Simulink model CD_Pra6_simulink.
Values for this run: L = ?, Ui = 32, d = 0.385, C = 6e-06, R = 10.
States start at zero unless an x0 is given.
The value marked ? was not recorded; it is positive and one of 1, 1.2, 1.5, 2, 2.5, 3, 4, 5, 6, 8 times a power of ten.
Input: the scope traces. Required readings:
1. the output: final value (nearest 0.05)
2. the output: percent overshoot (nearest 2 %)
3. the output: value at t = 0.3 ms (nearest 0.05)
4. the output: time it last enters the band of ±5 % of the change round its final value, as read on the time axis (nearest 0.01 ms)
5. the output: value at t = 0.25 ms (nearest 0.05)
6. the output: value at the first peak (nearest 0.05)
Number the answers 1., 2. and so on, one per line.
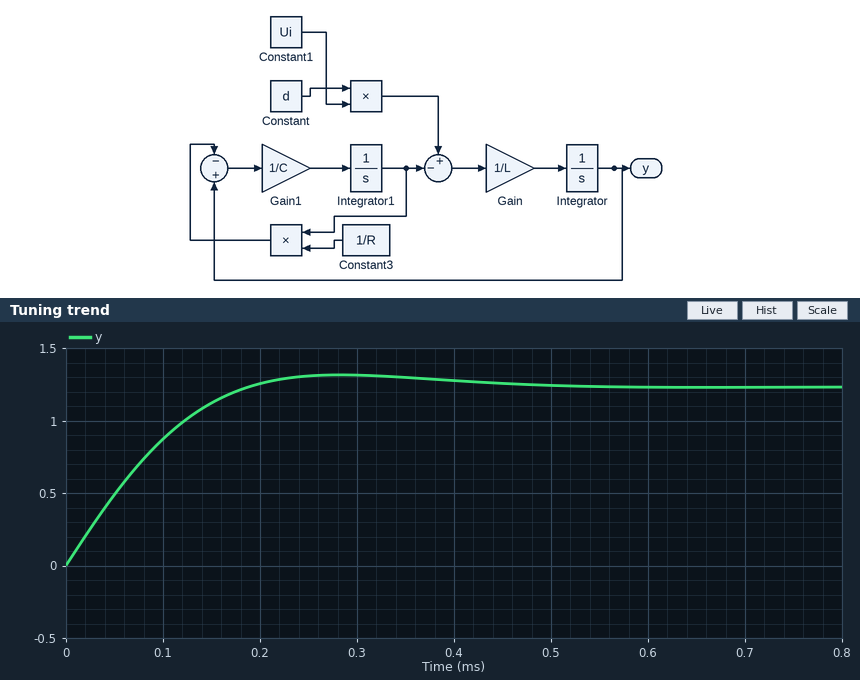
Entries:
1. 1.25
2. 6 %
3. 1.30
4. 0.36 ms
5. 1.30
6. 1.30
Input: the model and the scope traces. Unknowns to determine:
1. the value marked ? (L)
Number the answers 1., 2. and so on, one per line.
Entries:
1. 0.0012
